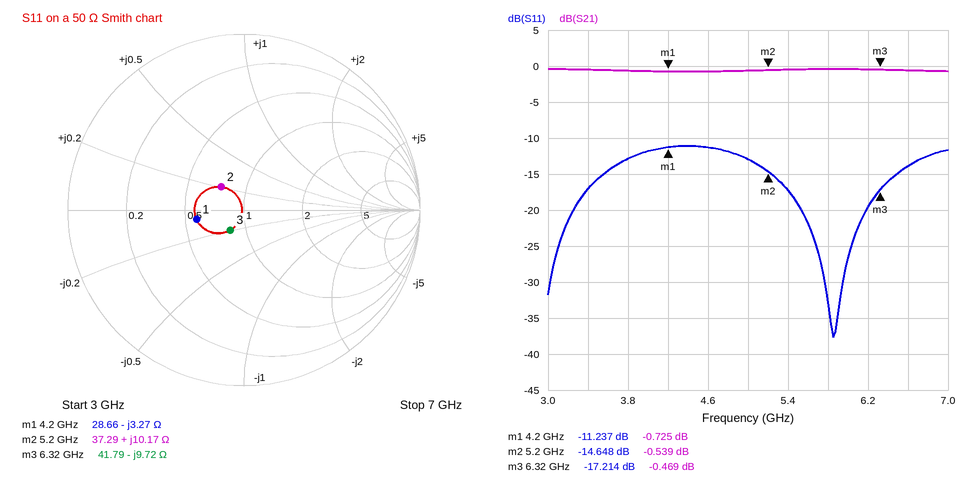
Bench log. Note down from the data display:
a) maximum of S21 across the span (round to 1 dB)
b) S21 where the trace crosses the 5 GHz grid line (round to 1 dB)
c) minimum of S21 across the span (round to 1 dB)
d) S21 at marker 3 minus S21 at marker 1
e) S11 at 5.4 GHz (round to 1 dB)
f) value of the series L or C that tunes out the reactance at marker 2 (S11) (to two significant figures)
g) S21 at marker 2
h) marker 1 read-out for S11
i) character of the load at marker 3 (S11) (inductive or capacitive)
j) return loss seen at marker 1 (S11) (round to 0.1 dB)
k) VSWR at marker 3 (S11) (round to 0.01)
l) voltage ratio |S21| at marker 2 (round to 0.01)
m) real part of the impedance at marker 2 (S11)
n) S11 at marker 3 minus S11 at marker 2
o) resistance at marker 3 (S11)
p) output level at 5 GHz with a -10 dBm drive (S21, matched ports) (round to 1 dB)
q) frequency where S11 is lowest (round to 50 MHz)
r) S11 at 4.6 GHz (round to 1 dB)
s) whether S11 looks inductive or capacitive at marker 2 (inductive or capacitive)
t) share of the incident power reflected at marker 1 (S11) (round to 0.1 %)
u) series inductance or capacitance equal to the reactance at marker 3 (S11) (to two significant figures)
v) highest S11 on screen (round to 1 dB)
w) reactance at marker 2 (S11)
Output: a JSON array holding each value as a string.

["0 dB", "-1 dB", "-1 dB", "0.256 dB", "-17 dB", "3.0 pF", "-0.539 dB", "-11.237 dB", "capacitive", "11.2 dB", "1.32", "0.94", "37.29 Ω", "-2.566 dB", "41.79 Ω", "-11 dBm", "5.85 GHz", "-11 dB", "inductive", "7.5 %", "2.6 pF", "-11 dB", "+10.17 Ω"]
